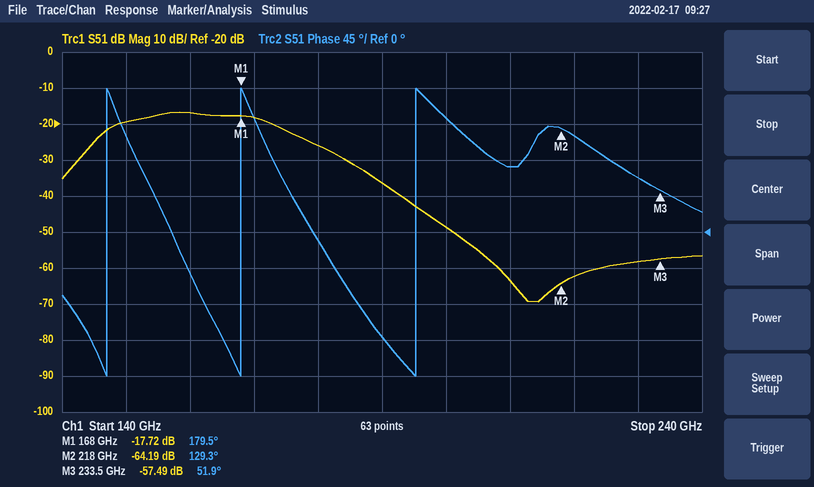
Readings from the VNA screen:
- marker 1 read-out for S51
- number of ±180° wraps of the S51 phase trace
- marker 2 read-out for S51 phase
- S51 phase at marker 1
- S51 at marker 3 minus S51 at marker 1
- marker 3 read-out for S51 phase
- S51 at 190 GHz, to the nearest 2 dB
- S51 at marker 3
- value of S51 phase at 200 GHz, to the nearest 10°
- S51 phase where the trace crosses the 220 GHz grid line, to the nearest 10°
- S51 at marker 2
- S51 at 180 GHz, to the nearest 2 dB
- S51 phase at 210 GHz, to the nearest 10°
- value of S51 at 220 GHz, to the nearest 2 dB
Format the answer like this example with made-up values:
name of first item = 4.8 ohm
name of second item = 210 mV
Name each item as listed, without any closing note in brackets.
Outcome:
marker 1 read-out for S51 = -17.72 dB
number of ±180° wraps of the S51 phase trace = 3
marker 2 read-out for S51 phase = 129.3°
S51 phase at marker 1 = 179.5°
S51 at marker 3 minus S51 at marker 1 = -39.77 dB
marker 3 read-out for S51 phase = 51.9°
S51 at 190 GHz, to the nearest 2 dB = -36 dB
S51 at marker 3 = -57.49 dB
value of S51 phase at 200 GHz, to the nearest 10° = 140°
S51 phase where the trace crosses the 220 GHz grid line, to the nearest 10° = 120°
S51 at marker 2 = -64.19 dB
S51 at 180 GHz, to the nearest 2 dB = -26 dB
S51 phase at 210 GHz, to the nearest 10° = 80°
value of S51 at 220 GHz, to the nearest 2 dB = -62 dB
